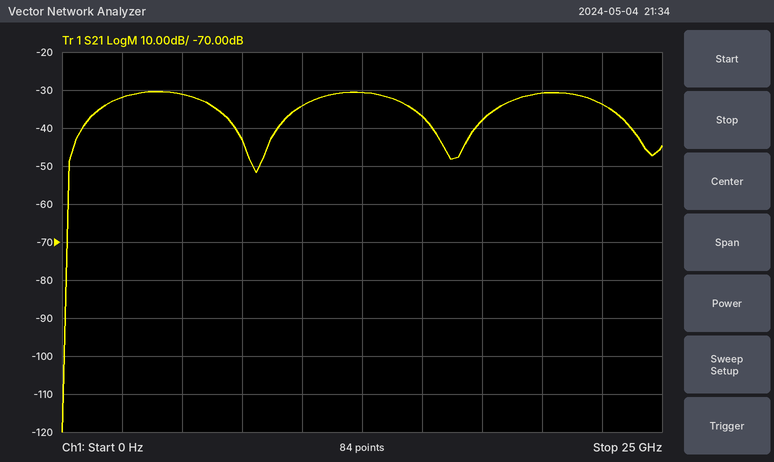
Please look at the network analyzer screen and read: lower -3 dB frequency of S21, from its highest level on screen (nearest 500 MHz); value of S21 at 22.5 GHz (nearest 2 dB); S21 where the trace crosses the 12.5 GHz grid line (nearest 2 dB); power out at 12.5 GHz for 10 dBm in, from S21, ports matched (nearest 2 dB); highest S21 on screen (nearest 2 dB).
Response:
2.0 GHz
-34 dB
-30 dB
-20 dBm
-30 dB
